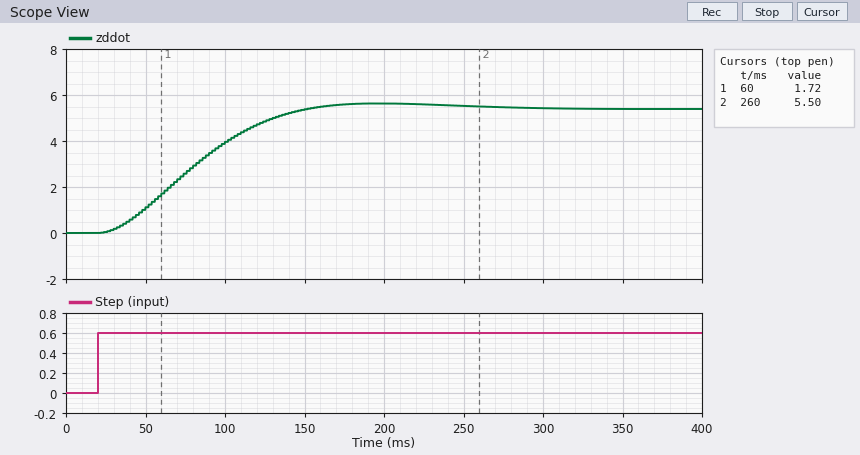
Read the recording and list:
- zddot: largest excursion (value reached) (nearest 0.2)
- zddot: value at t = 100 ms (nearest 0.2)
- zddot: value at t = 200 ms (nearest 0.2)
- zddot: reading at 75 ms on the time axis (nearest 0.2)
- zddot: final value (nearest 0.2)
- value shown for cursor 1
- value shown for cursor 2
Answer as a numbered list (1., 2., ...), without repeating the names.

1. 5.6
2. 4.0
3. 5.6
4. 2.6
5. 5.4
6. 1.72
7. 5.50
